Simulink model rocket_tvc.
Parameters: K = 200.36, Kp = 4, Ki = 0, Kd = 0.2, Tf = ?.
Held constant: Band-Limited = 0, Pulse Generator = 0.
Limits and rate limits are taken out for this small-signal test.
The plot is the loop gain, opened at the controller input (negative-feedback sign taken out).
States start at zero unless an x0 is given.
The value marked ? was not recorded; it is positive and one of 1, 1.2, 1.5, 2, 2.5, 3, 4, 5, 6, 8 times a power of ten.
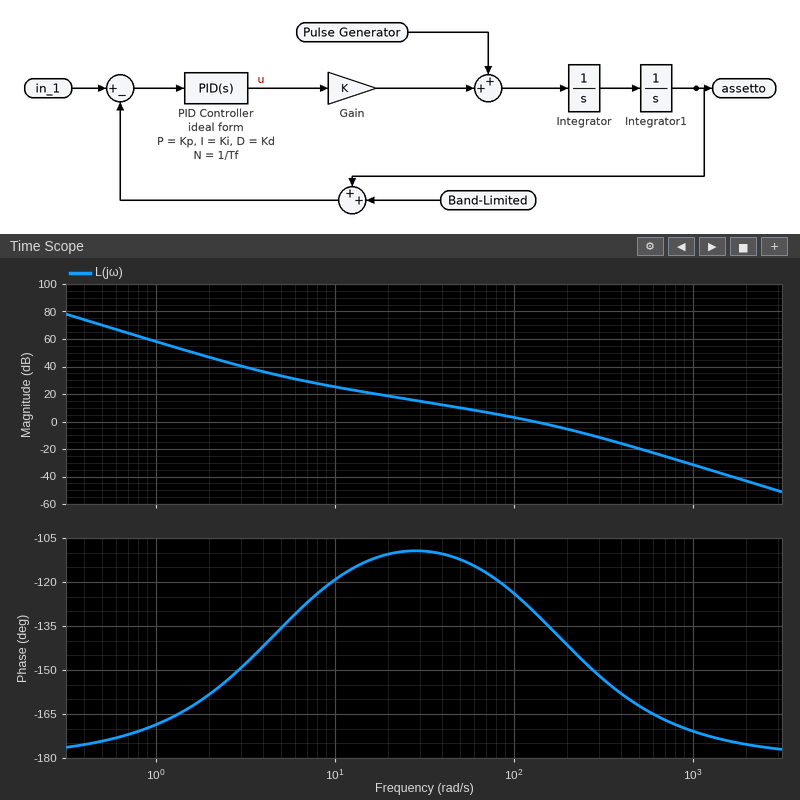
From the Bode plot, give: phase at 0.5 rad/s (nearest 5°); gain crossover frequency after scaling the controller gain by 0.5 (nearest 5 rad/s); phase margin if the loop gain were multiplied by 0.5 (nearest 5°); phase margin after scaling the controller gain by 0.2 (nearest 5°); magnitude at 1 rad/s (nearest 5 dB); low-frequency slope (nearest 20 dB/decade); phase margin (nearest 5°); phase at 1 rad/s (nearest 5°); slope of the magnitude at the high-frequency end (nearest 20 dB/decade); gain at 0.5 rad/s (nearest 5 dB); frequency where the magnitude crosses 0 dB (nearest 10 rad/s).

-175°
75 rad/s
60°
70°
60 dB
-40 dB/decade
50°
-170°
-40 dB/decade
70 dB
130 rad/s
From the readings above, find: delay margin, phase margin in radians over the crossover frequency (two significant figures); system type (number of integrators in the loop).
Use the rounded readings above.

0.0067 s
2
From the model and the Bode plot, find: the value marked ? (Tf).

0.006
